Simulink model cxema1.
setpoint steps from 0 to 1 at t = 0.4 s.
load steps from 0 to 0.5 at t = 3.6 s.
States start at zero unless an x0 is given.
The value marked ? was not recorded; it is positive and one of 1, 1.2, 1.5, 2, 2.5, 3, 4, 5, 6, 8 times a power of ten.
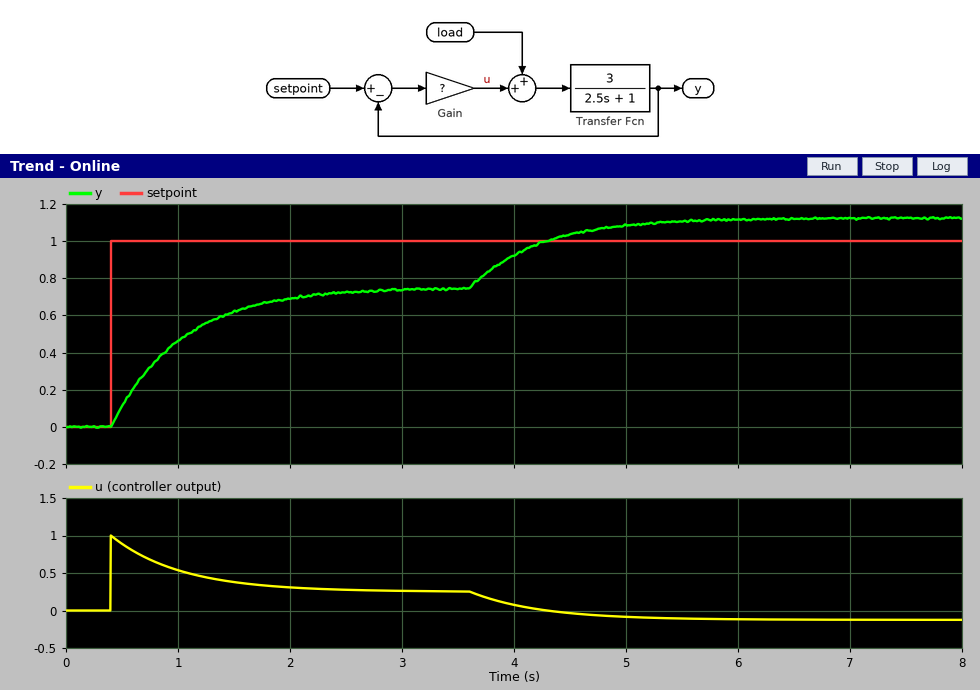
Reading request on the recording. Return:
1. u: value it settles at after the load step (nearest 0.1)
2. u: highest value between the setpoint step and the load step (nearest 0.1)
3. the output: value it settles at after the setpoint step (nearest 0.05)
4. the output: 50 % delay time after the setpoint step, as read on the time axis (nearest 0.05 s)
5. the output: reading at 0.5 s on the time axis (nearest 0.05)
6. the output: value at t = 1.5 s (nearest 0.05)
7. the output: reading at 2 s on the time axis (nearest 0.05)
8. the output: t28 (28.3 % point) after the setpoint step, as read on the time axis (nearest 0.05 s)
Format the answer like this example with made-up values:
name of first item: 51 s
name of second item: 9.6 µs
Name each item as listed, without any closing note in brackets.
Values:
u: value it settles at after the load step: -0.1
u: highest value between the setpoint step and the load step: 1.0
the output: value it settles at after the setpoint step: 0.75
the output: 50 % delay time after the setpoint step, as read on the time axis: 0.85 s
the output: reading at 0.5 s on the time axis: 0.10
the output: value at t = 1.5 s: 0.60
the output: reading at 2 s on the time axis: 0.70
the output: t28 (28.3 % point) after the setpoint step, as read on the time axis: 0.60 s
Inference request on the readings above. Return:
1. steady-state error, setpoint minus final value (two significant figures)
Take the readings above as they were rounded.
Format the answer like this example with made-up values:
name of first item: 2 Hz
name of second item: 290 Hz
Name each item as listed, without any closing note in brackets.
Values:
steady-state error, setpoint minus final value: 0.25
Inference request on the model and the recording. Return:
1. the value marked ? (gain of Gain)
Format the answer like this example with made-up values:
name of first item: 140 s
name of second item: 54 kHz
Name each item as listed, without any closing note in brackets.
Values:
the value marked ?: 1
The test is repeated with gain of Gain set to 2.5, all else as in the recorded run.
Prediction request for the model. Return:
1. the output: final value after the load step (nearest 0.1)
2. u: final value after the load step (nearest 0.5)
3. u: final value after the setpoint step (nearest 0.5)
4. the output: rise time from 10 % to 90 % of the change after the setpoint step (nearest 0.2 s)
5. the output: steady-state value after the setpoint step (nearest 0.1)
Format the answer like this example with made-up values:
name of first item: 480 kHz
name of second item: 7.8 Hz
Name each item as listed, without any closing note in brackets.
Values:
the output: final value after the load step: 1.1
u: final value after the load step: 0.0
u: final value after the setpoint step: 0.5
the output: rise time from 10 % to 90 % of the change after the setpoint step: 0.6 s
the output: steady-state value after the setpoint step: 0.9
